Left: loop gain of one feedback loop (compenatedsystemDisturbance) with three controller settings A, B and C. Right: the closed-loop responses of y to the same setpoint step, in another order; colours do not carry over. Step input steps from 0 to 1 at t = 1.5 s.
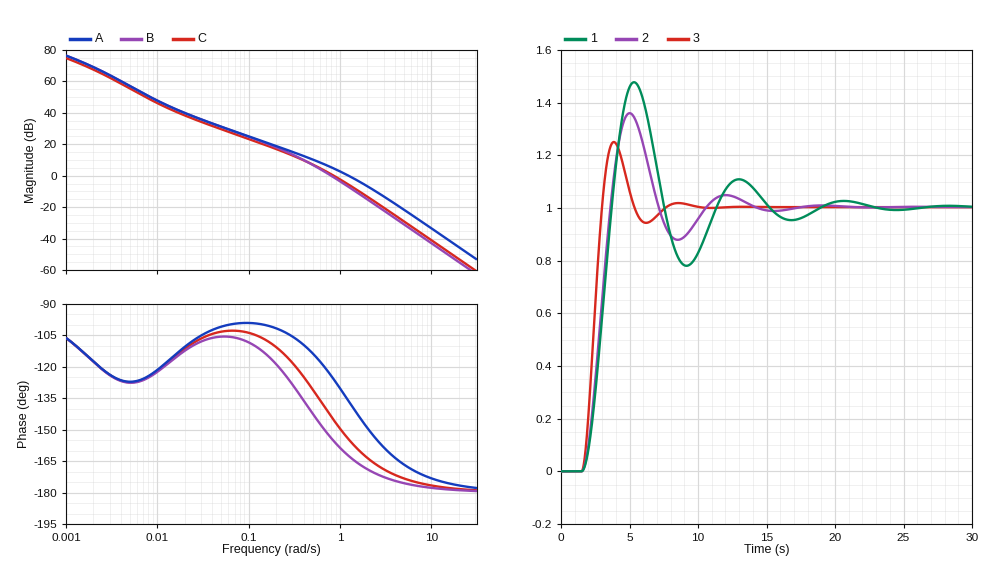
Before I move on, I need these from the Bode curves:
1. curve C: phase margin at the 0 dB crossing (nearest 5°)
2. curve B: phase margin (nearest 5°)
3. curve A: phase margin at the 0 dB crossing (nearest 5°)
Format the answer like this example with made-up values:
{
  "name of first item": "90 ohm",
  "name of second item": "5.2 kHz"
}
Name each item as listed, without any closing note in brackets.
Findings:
{
  "curve C: phase margin at the 0 dB crossing": "35°",
  "curve B: phase margin": "25°",
  "curve A: phase margin at the 0 dB crossing": "45°"
}
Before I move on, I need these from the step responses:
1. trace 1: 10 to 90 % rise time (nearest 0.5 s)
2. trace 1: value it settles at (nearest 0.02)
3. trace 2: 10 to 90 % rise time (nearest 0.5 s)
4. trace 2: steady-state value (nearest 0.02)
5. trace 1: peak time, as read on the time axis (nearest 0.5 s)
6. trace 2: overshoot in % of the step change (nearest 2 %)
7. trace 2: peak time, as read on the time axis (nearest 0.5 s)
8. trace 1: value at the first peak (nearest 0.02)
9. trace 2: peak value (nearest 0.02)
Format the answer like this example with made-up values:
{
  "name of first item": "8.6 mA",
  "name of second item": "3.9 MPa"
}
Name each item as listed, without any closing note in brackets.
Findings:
{
  "trace 1: 10 to 90 % rise time": "1.5 s",
  "trace 1: value it settles at": "1.00",
  "trace 2: 10 to 90 % rise time": "1.5 s",
  "trace 2: steady-state value": "1.00",
  "trace 1: peak time, as read on the time axis": "5.5 s",
  "trace 2: overshoot in % of the step change": "36 %",
  "trace 2: peak time, as read on the time axis": "5.0 s",
  "trace 1: value at the first peak": "1.48",
  "trace 2: peak value": "1.36"
}
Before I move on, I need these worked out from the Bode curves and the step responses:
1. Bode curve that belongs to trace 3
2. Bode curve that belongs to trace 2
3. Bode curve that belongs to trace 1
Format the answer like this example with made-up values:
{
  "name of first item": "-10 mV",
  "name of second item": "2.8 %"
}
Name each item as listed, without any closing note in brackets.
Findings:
{
  "Bode curve that belongs to trace 3": "A",
  "Bode curve that belongs to trace 2": "C",
  "Bode curve that belongs to trace 1": "B"
}
